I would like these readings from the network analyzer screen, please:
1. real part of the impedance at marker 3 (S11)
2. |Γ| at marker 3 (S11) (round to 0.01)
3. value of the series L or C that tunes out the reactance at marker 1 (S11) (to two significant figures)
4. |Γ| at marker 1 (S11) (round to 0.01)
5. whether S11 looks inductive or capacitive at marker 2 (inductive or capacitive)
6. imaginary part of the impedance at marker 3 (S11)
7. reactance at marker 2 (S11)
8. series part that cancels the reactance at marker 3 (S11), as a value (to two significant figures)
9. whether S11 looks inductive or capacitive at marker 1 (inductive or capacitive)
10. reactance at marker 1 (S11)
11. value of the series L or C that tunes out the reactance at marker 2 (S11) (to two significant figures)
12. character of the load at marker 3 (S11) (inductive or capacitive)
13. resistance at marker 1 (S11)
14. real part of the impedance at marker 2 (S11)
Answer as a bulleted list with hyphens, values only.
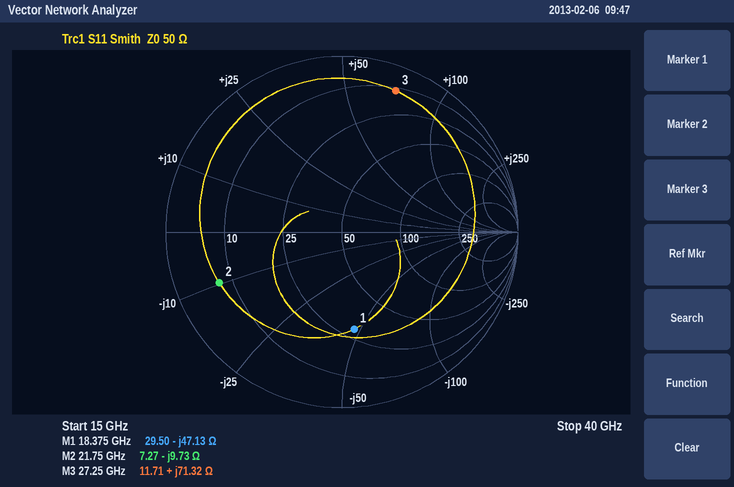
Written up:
- 11.71 Ω
- 0.86
- 410 pH
- 0.56
- capacitive
- +71.32 Ω
- -9.73 Ω
- 82 fF
- capacitive
- -47.13 Ω
- 71 pH
- inductive
- 29.50 Ω
- 7.27 Ω
